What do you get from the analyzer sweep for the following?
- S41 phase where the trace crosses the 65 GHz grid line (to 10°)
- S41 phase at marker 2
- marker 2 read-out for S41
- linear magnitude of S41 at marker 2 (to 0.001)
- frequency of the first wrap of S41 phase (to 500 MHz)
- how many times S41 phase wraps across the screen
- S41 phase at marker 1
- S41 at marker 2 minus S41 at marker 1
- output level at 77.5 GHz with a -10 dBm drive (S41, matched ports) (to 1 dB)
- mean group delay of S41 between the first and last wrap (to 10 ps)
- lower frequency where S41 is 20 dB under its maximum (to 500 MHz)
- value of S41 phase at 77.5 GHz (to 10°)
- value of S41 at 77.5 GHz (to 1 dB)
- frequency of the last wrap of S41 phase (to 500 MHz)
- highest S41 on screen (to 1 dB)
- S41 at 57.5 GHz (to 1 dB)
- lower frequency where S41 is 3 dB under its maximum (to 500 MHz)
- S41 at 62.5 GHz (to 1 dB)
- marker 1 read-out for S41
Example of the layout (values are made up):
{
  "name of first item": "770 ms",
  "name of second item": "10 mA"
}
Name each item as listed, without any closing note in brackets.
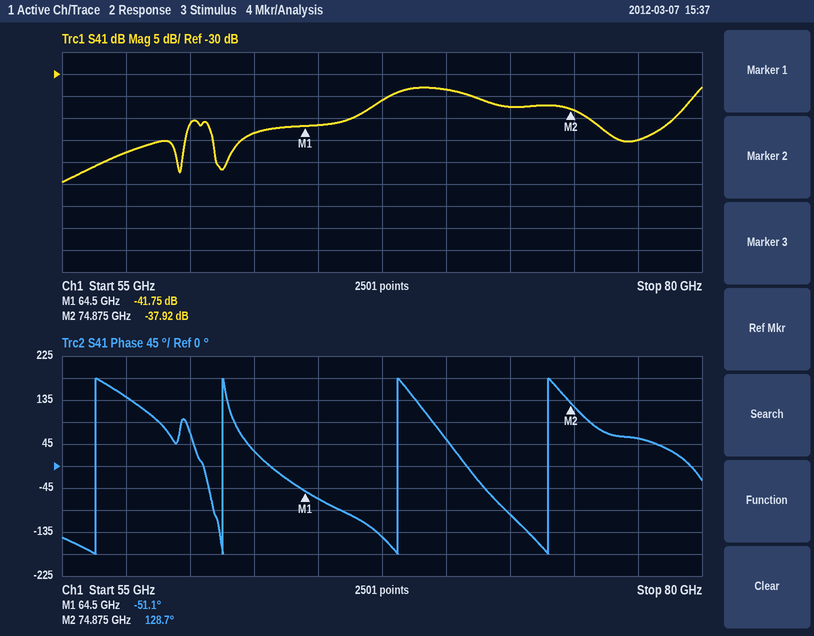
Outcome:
{
  "S41 phase where the trace crosses the 65 GHz grid line": "-70°",
  "S41 phase at marker 2": "128.7°",
  "marker 2 read-out for S41": "-37.92 dB",
  "linear magnitude of S41 at marker 2": "0.013",
  "frequency of the first wrap of S41 phase": "56.5 GHz",
  "how many times S41 phase wraps across the screen": "4",
  "S41 phase at marker 1": "-51.1°",
  "S41 at marker 2 minus S41 at marker 1": "3.83 dB",
  "output level at 77.5 GHz with a -10 dBm drive (S41, matched ports)": "-55 dBm",
  "mean group delay of S41 between the first and last wrap": "170 ps",
  "lower frequency where S41 is 20 dB under its maximum": "55.5 GHz",
  "value of S41 phase at 77.5 GHz": "60°",
  "value of S41 at 77.5 GHz": "-45 dB",
  "frequency of the last wrap of S41 phase": "74.0 GHz",
  "highest S41 on screen": "-33 dB",
  "S41 at 57.5 GHz": "-48 dB",
  "lower frequency where S41 is 3 dB under its maximum": "67.5 GHz",
  "S41 at 62.5 GHz": "-43 dB",
  "marker 1 read-out for S41": "-41.75 dB"
}
